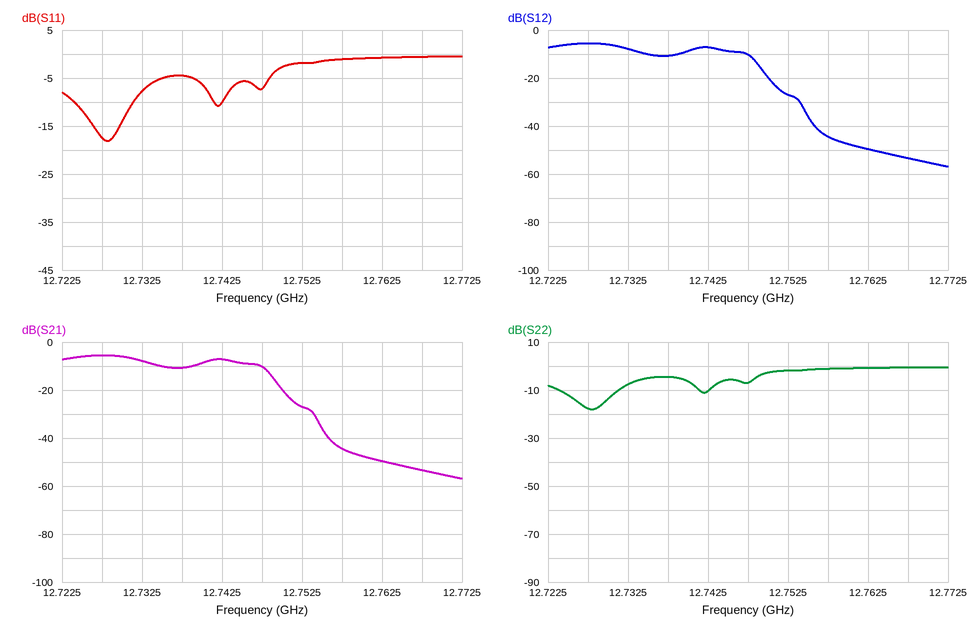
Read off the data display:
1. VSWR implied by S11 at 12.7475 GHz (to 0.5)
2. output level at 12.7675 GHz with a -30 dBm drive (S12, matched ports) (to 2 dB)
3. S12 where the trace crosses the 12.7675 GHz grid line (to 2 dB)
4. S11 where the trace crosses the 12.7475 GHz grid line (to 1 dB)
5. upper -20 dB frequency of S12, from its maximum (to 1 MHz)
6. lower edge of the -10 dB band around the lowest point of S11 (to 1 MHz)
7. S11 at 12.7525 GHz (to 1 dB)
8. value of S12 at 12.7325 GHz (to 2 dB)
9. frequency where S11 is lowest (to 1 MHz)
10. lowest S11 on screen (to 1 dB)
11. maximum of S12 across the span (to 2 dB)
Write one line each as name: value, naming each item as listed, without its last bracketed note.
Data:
VSWR implied by S11 at 12.7475 GHz: 2.5
output level at 12.7675 GHz with a -30 dBm drive (S12, matched ports): -84 dBm
S12 where the trace crosses the 12.7675 GHz grid line: -54 dB
S11 where the trace crosses the 12.7475 GHz grid line: -7 dB
upper -20 dB frequency of S12, from its maximum: 12.752 GHz
lower edge of the -10 dB band around the lowest point of S11: 12.724 GHz
S11 at 12.7525 GHz: -2 dB
value of S12 at 12.7325 GHz: -8 dB
frequency where S11 is lowest: 12.728 GHz
lowest S11 on screen: -18 dB
maximum of S12 across the span: -6 dB
